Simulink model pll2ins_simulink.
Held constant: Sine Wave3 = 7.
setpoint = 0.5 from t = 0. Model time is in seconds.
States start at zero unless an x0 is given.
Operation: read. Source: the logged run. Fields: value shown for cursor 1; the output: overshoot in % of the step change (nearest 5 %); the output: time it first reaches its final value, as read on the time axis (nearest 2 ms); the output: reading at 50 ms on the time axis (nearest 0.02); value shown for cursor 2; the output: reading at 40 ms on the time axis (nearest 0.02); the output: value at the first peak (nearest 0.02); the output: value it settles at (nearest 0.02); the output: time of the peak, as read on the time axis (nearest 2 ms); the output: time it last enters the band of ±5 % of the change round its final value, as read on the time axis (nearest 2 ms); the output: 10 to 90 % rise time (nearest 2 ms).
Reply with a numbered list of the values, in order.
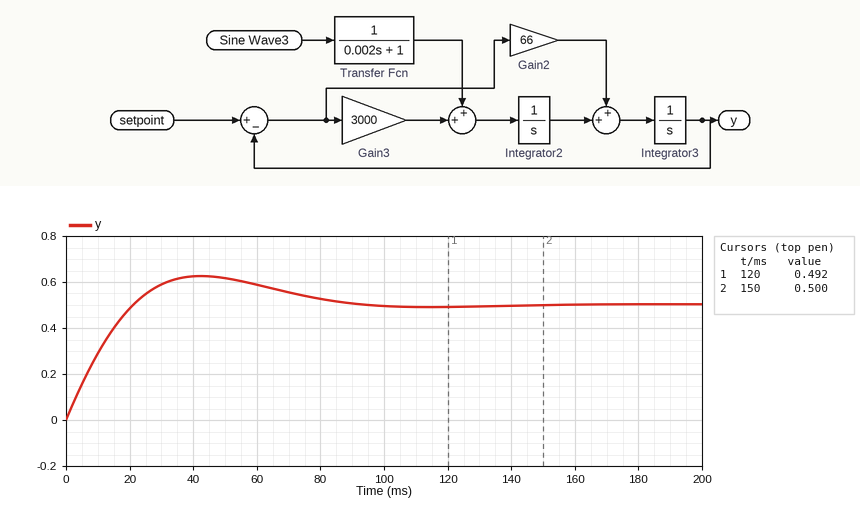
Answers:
1. 0.492
2. 25 %
3. 22 ms
4. 0.62
5. 0.500
6. 0.62
7. 0.62
8. 0.50
9. 42 ms
10. 80 ms
11. 16 ms
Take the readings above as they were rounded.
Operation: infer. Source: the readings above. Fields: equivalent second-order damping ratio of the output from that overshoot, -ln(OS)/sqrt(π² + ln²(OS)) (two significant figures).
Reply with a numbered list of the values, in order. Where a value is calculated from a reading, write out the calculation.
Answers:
1. ln(0.25) = -1.386; 1.386 / sqrt(9.870 + 1.922) = 0.40
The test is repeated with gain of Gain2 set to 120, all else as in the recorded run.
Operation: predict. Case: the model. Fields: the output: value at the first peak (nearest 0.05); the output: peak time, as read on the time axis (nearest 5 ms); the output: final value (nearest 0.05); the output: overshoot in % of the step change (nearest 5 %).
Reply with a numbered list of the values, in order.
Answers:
1. 0.55
2. 35 ms
3. 0.50
4. 10 %
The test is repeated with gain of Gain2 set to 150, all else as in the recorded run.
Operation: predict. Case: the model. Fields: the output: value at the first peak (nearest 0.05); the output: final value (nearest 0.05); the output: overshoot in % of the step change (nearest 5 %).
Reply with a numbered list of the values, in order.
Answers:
1. 0.55
2. 0.50
3. 10 %
